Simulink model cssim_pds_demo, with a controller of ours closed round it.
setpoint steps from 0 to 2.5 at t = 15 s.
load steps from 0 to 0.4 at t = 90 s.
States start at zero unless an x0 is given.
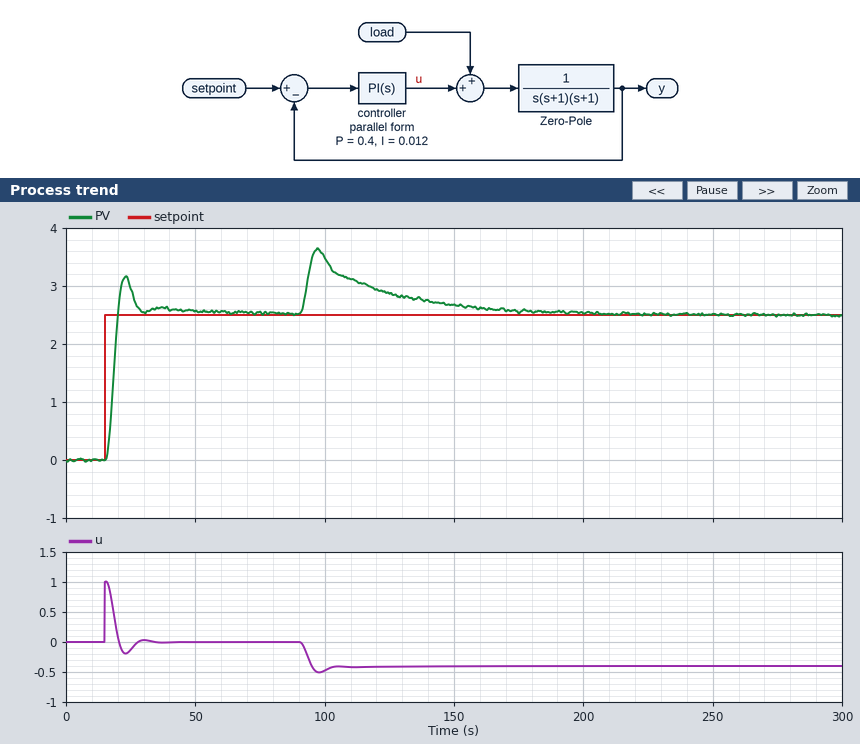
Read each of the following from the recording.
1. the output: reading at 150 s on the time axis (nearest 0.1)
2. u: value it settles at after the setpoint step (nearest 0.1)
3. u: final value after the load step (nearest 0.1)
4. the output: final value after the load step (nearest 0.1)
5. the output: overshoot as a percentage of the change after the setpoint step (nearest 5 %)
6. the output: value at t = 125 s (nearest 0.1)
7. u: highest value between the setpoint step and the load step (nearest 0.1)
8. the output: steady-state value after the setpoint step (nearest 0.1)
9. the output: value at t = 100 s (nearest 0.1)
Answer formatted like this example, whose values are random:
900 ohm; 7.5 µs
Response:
2.7; 0.0; -0.4; 2.5; 25 %; 2.9; 1.0; 2.5; 3.5
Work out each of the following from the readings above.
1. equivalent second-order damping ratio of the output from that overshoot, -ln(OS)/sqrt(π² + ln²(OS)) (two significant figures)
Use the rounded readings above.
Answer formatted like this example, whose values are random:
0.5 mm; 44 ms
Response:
0.40
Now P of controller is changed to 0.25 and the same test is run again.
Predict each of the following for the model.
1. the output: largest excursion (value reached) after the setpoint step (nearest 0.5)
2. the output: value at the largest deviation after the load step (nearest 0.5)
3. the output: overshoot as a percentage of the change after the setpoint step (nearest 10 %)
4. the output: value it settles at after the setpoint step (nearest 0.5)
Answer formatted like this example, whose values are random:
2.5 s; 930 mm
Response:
3.0; 4.0; 20 %; 2.5
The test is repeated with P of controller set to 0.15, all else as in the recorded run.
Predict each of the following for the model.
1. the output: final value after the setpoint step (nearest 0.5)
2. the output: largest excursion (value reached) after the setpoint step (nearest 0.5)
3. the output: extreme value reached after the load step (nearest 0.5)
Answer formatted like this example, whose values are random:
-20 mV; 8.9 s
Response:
2.5; 3.5; 4.5
